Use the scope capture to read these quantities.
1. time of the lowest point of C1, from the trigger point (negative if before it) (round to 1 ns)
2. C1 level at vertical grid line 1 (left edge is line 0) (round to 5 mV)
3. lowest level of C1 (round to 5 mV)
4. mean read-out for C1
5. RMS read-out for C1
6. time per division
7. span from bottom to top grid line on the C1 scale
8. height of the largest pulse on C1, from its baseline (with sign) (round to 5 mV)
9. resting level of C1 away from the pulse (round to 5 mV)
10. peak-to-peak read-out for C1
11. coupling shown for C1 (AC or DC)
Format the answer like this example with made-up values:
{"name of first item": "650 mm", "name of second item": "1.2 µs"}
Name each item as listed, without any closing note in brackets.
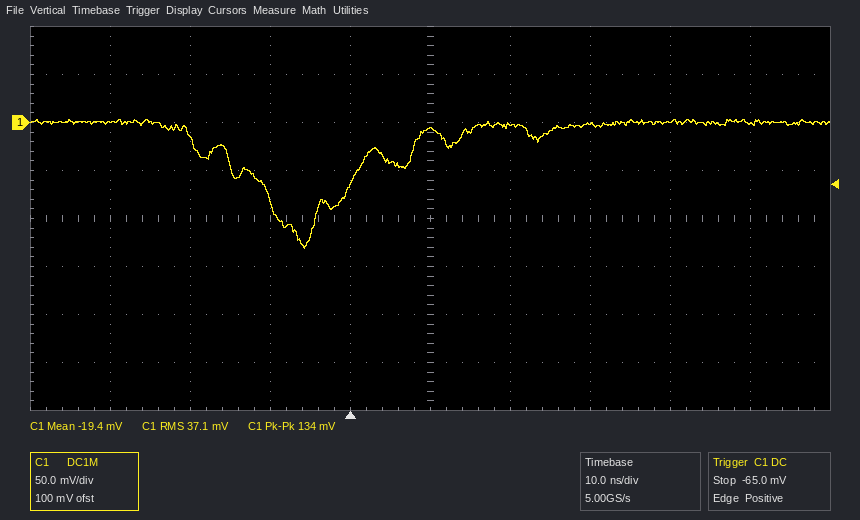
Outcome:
{"time of the lowest point of C1, from the trigger point (negative if before it)": "-6 ns", "C1 level at vertical grid line 1 (left edge is line 0)": "0 mV", "lowest level of C1": "-130 mV", "mean read-out for C1": "-19.4 mV", "RMS read-out for C1": "37.1 mV", "time per division": "10 ns", "span from bottom to top grid line on the C1 scale": "400 mV", "height of the largest pulse on C1, from its baseline (with sign)": "-130 mV", "resting level of C1 away from the pulse": "0 mV", "peak-to-peak read-out for C1": "134 mV", "coupling shown for C1": "DC"}
